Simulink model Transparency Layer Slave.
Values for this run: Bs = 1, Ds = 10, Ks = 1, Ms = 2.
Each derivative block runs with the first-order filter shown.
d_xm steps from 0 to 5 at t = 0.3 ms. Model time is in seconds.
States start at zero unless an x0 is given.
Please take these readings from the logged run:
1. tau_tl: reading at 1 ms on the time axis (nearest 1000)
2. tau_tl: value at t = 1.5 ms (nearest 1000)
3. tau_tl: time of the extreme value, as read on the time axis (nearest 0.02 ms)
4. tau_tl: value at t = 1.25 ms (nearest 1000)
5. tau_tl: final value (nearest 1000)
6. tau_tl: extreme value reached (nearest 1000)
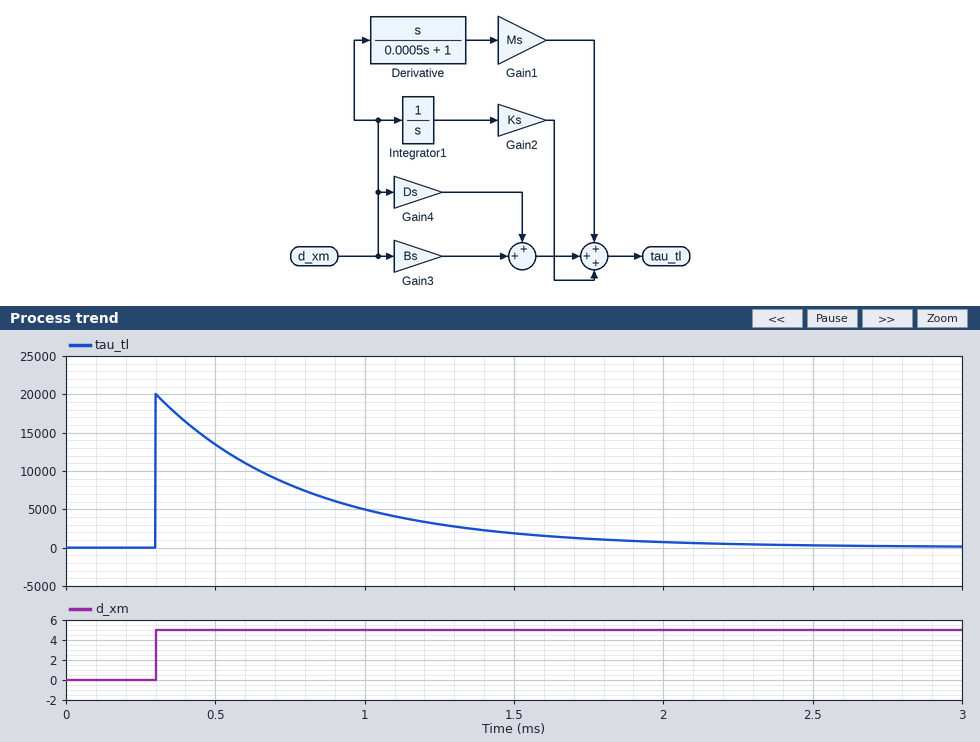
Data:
5000
2000
0.30 ms
3000
0
20000
